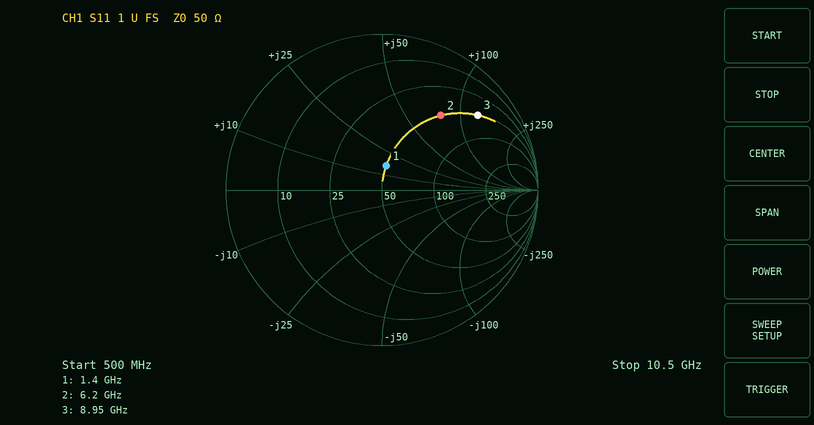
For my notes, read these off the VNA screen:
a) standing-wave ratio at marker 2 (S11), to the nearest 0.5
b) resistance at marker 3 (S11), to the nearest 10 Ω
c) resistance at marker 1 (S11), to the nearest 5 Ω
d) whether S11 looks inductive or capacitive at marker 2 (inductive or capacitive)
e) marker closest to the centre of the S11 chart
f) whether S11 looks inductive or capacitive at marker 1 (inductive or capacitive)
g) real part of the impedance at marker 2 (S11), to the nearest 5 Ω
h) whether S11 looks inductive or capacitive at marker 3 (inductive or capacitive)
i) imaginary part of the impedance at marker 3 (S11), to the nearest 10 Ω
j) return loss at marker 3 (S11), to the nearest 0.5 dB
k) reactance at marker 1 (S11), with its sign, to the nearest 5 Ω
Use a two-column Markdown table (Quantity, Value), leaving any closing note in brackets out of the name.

| Quantity | Value |
|---|---|
| standing-wave ratio at marker 2 (S11), to the nearest 0.5 | 4.0 |
| resistance at marker 3 (S11), to the nearest 10 Ω | 50 Ω |
| resistance at marker 1 (S11), to the nearest 5 Ω | 50 Ω |
| whether S11 looks inductive or capacitive at marker 2 | inductive |
| marker closest to the centre of the S11 chart | marker 1 |
| whether S11 looks inductive or capacitive at marker 1 | inductive |
| real part of the impedance at marker 2 (S11), to the nearest 5 Ω | 50 Ω |
| whether S11 looks inductive or capacitive at marker 3 | inductive |
| imaginary part of the impedance at marker 3 (S11), to the nearest 10 Ω | +130 Ω |
| return loss at marker 3 (S11), to the nearest 0.5 dB | 2.0 dB |
| reactance at marker 1 (S11), with its sign, to the nearest 5 Ω | +15 Ω |
